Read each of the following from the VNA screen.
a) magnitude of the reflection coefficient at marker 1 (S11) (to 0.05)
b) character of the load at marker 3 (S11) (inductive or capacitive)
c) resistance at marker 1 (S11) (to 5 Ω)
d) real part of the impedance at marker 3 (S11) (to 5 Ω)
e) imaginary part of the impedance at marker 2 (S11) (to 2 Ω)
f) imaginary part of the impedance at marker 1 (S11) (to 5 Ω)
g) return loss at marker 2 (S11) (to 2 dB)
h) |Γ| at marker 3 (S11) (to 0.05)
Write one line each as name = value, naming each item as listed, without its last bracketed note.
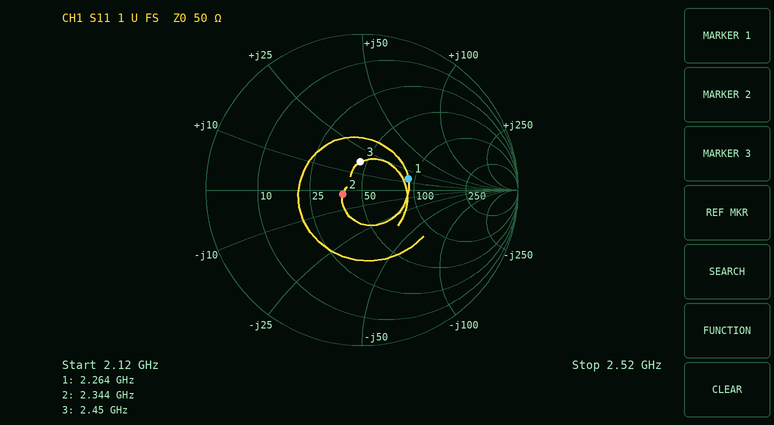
magnitude of the reflection coefficient at marker 1 (S11) = 0.30
character of the load at marker 3 (S11) = inductive
resistance at marker 1 (S11) = 90 Ω
real part of the impedance at marker 3 (S11) = 45 Ω
imaginary part of the impedance at marker 2 (S11) = -2 Ω
imaginary part of the impedance at marker 1 (S11) = +15 Ω
return loss at marker 2 (S11) = 18 dB
|Γ| at marker 3 (S11) = 0.20
